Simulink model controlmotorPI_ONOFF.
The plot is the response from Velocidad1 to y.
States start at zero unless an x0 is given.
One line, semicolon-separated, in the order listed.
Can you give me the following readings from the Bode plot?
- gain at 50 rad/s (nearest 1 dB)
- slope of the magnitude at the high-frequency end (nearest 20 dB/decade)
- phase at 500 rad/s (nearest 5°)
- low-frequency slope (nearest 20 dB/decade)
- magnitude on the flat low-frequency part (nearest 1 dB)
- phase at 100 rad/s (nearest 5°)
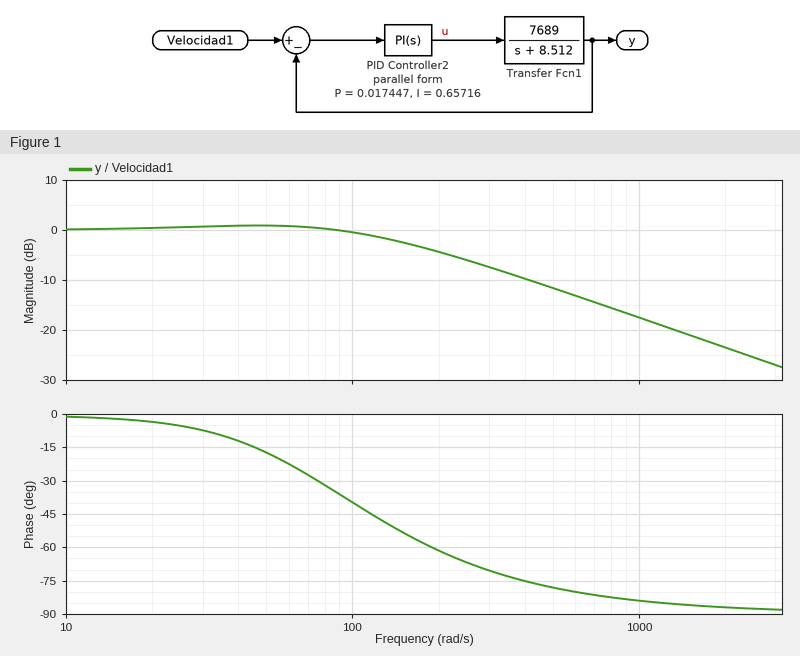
1 dB; -20 dB/decade; -80°; 0 dB/decade; 0 dB; -40°
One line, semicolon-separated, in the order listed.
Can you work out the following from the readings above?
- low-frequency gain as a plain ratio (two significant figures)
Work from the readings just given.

1.0
